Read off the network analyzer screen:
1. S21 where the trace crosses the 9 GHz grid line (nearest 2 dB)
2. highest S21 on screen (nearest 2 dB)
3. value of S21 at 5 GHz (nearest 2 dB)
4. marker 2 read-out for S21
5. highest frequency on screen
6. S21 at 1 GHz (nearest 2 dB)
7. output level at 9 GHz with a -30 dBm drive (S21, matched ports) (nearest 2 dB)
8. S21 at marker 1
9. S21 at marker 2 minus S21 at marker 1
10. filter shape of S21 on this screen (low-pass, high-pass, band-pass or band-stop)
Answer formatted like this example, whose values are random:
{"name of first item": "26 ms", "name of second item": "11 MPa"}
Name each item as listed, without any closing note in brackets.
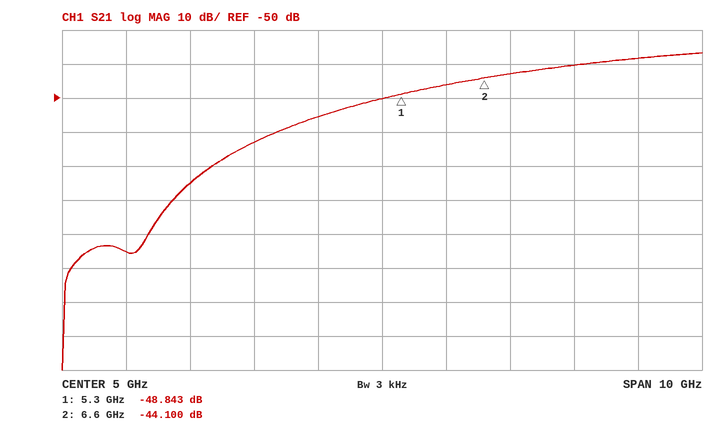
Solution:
{"S21 where the trace crosses the 9 GHz grid line": "-38 dB", "highest S21 on screen": "-36 dB", "value of S21 at 5 GHz": "-50 dB", "marker 2 read-out for S21": "-44.100 dB", "highest frequency on screen": "10 GHz", "S21 at 1 GHz": "-96 dB", "output level at 9 GHz with a -30 dBm drive (S21, matched ports)": "-68 dBm", "S21 at marker 1": "-48.843 dB", "S21 at marker 2 minus S21 at marker 1": "4.743 dB", "filter shape of S21 on this screen": "high-pass"}
